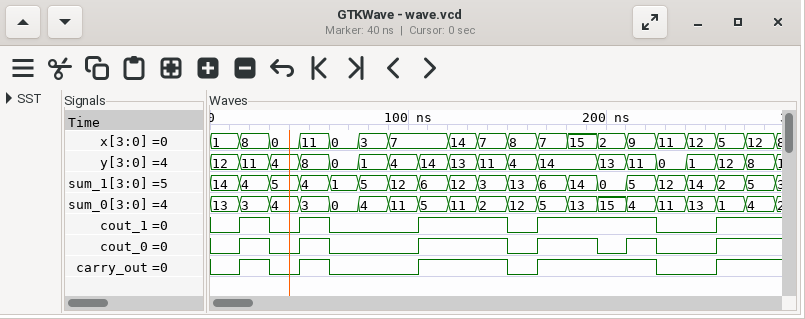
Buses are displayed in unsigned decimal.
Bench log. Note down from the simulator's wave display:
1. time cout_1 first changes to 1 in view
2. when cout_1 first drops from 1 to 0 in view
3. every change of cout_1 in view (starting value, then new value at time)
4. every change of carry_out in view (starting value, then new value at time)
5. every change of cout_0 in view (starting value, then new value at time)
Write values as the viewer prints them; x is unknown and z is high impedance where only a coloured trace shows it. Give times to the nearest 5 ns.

15 ns
30 ns
0, 1 at 15 ns, 0 at 30 ns, 1 at 45 ns, 0 at 60 ns, 1 at 105 ns, 0 at 150 ns, 1 at 165 ns, 0 at 225 ns, 1 at 255 ns
0, 1 at 15 ns, 0 at 30 ns, 1 at 45 ns, 0 at 60 ns, 1 at 105 ns, 0 at 150 ns, 1 at 165 ns, 0 at 225 ns, 1 at 255 ns
0, 1 at 15 ns, 0 at 30 ns, 1 at 45 ns, 0 at 60 ns, 1 at 105 ns, 0 at 150 ns, 1 at 165 ns, 0 at 195 ns, 1 at 210 ns, 0 at 225 ns, 1 at 255 ns
